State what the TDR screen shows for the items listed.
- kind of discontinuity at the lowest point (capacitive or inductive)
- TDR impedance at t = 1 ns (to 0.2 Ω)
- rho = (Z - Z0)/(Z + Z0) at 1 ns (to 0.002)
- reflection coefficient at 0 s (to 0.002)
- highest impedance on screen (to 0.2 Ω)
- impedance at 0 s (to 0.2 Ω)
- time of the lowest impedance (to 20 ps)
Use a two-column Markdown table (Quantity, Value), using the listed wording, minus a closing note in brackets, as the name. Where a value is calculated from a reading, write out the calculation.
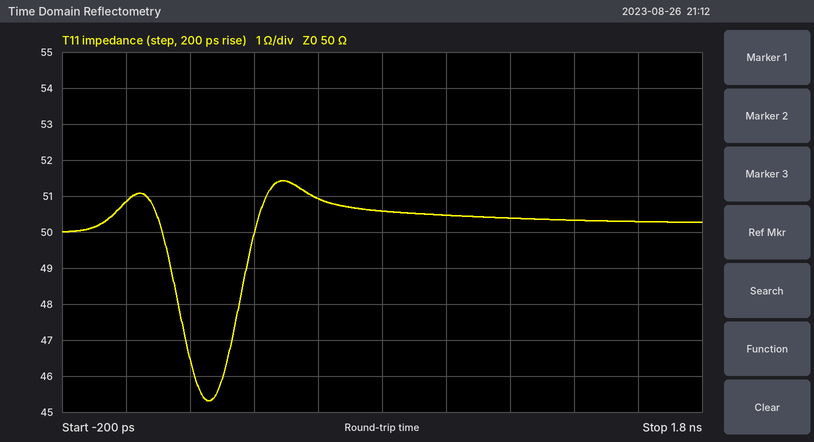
| Quantity | Value |
|---|---|
| kind of discontinuity at the lowest point | capacitive |
| TDR impedance at t = 1 ns | 50.4 Ω |
| rho = (Z - Z0)/(Z + Z0) at 1 ns | (50.4 − 50)/(50.4 + 50) ≈ +0.004 |
| reflection coefficient at 0 s | (50.8 − 50)/(50.8 + 50) ≈ +0.008 |
| highest impedance on screen | 51.4 Ω |
| impedance at 0 s | 50.8 Ω |
| time of the lowest impedance | 260 ps |
